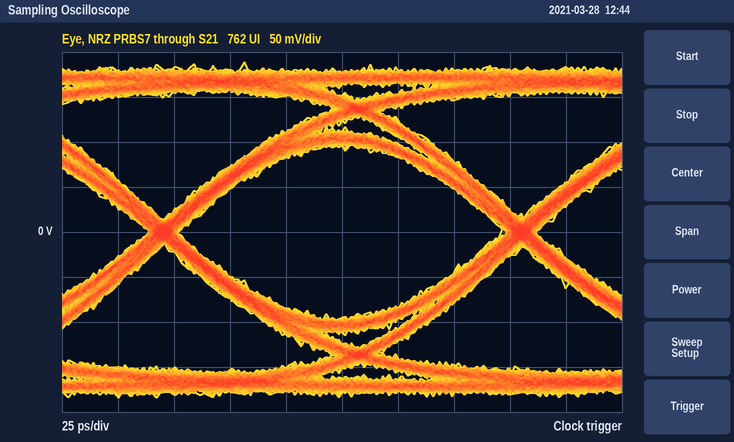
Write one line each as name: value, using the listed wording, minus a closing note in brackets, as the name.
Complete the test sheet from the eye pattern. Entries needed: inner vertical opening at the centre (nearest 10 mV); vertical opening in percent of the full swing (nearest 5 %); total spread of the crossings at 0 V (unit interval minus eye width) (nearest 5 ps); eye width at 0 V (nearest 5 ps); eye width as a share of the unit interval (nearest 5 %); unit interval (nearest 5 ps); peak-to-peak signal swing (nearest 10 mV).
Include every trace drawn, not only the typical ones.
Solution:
inner vertical opening at the centre: 190 mV
vertical opening in percent of the full swing: 50 %
total spread of the crossings at 0 V (unit interval minus eye width): 15 ps
eye width at 0 V: 145 ps
eye width as a share of the unit interval: 90 %
unit interval: 160 ps
peak-to-peak signal swing: 370 mV
